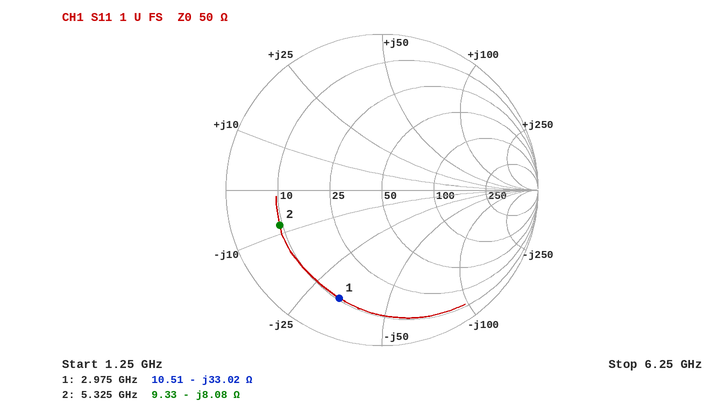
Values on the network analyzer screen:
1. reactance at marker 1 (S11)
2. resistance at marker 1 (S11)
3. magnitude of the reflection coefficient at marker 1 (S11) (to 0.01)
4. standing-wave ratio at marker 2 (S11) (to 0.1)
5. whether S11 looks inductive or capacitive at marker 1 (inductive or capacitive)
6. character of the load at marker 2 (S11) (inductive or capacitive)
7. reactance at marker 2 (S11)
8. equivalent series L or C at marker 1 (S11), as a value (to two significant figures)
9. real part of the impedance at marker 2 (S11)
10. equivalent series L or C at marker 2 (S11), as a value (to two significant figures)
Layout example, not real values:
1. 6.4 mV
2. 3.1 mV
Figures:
1. -33.02 Ω
2. 10.51 Ω
3. 0.75
4. 5.5
5. capacitive
6. capacitive
7. -8.08 Ω
8. 1.6 pF
9. 9.33 Ω
10. 3.7 pF
